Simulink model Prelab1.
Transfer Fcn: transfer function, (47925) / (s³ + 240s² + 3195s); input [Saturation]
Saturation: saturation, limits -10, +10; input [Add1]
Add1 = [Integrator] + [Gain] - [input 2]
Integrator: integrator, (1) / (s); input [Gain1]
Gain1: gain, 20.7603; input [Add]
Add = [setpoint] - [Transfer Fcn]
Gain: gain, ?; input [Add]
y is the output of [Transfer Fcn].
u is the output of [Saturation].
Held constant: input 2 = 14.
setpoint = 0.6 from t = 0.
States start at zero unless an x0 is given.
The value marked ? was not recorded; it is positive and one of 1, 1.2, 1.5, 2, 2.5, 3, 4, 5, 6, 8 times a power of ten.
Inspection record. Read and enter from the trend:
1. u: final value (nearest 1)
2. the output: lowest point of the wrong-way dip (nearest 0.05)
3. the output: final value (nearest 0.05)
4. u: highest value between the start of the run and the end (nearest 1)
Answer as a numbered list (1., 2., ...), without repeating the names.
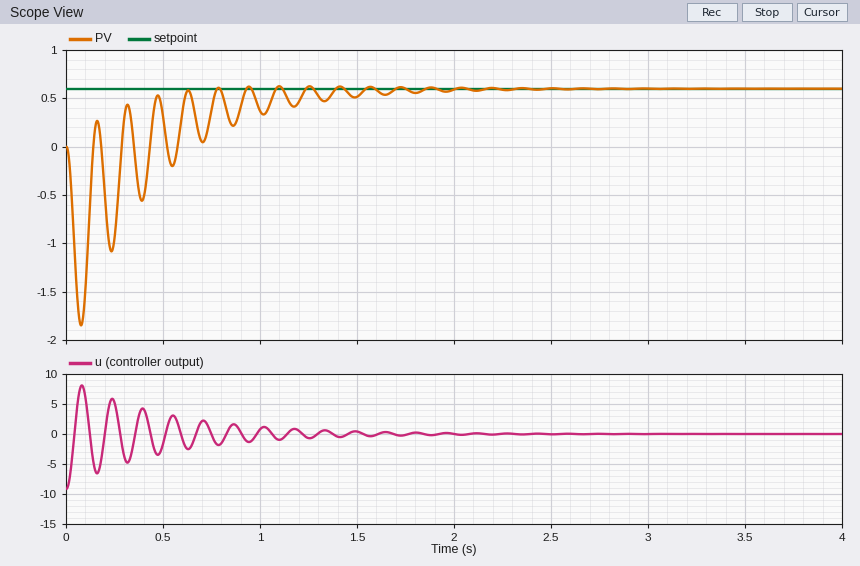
1. 0
2. -1.85
3. 0.60
4. 8
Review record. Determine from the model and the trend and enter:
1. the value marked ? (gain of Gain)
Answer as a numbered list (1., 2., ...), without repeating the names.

1. 8
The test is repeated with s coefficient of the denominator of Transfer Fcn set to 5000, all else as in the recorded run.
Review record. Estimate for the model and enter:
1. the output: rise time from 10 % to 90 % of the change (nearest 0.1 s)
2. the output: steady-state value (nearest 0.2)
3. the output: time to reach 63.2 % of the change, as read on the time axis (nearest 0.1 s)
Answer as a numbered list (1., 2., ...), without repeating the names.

1. 0.8 s
2. 0.6
3. 0.8 s
